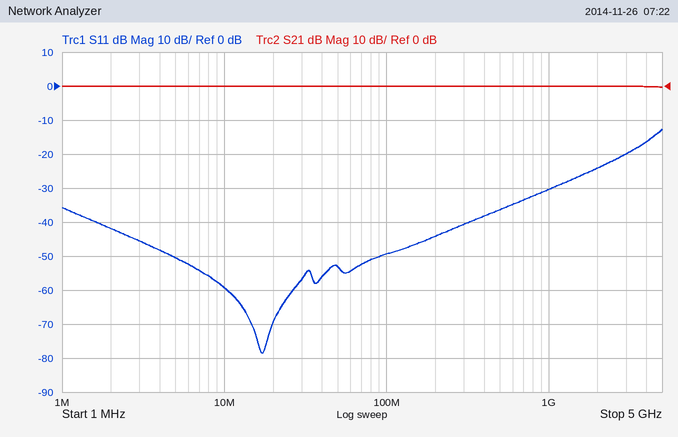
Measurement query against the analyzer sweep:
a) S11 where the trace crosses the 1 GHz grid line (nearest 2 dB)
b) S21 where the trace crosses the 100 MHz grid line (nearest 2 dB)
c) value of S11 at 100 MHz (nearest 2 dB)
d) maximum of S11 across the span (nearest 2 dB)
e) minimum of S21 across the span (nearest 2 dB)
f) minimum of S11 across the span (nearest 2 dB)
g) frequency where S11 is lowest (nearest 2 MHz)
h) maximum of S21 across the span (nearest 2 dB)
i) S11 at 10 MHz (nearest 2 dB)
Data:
-30 dB
0 dB
-50 dB
-12 dB
0 dB
-78 dB
18 MHz
0 dB
-60 dB
